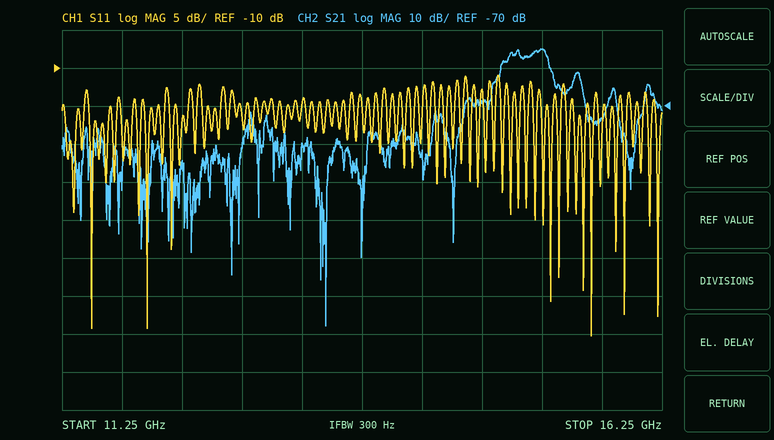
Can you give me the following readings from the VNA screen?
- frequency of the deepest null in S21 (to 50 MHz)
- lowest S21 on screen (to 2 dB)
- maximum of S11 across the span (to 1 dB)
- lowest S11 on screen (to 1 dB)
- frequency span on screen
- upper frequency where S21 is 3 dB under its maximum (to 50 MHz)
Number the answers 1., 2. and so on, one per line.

1. 13.45 GHz
2. -128 dB
3. -11 dB
4. -45 dB
5. 5 GHz
6. 15.30 GHz
